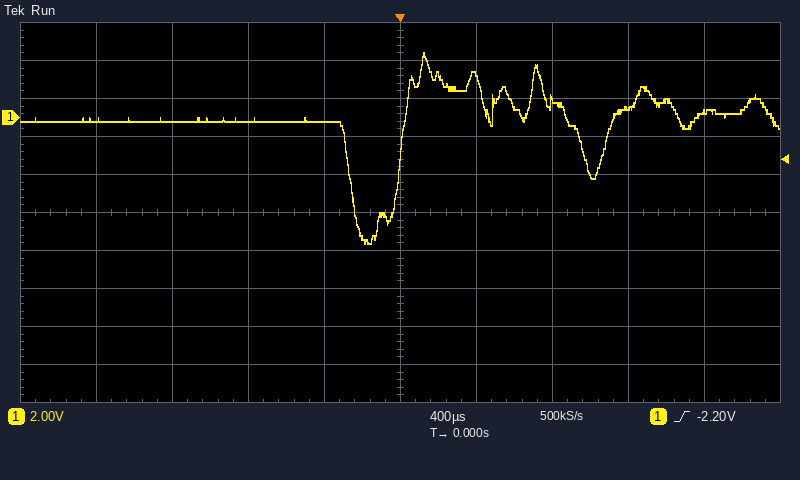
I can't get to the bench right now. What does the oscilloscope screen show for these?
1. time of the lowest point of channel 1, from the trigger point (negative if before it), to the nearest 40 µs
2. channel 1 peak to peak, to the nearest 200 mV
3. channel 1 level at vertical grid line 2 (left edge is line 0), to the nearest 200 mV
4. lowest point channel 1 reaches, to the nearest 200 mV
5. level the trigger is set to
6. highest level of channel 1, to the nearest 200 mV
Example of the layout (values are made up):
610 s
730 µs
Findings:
-160 µs
10.0 V
-200 mV
-6.6 V
-2.20 V
3.4 V
